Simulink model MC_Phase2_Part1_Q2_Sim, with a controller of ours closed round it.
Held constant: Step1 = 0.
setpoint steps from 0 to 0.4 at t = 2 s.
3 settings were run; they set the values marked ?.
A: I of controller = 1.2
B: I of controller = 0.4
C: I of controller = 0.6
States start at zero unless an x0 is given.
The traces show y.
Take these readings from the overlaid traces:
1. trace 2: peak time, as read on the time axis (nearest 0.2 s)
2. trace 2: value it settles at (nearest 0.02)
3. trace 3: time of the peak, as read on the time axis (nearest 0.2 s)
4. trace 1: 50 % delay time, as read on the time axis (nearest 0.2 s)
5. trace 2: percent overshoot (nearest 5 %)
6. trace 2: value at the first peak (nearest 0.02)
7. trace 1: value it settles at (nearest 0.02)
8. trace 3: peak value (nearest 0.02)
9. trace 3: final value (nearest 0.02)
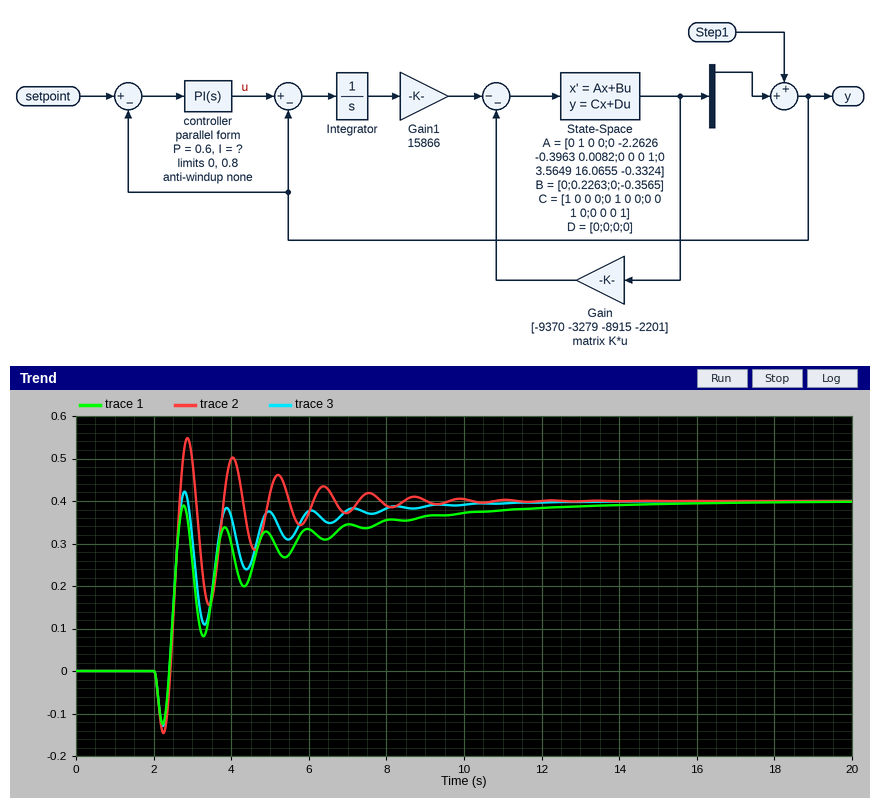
2.8 s
0.40
2.8 s
2.6 s
35 %
0.54
0.40
0.42
0.40
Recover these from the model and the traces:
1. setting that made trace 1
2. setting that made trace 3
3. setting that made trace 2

B
C
A
